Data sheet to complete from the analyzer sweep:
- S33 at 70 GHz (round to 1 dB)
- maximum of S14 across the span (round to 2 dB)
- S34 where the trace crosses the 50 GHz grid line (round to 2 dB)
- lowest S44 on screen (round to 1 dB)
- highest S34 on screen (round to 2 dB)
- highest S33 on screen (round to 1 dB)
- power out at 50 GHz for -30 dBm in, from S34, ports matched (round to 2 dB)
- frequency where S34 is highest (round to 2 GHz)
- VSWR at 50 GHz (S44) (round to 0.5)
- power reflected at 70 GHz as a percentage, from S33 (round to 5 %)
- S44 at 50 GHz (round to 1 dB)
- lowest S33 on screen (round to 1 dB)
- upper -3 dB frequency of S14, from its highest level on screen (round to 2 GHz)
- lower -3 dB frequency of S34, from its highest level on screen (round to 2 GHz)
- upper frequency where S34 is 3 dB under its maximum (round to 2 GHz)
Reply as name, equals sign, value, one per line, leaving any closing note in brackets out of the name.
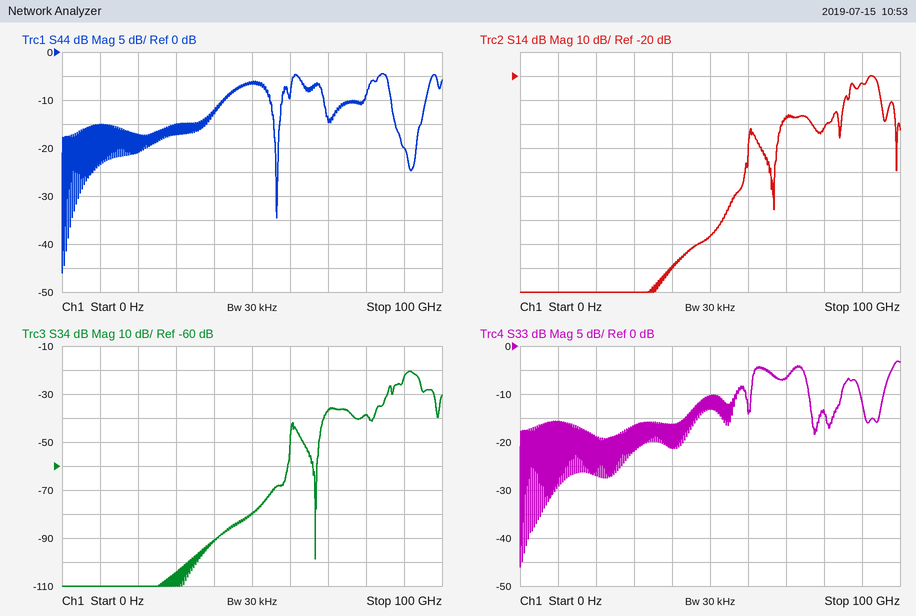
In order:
S33 at 70 GHz = -7 dB
maximum of S14 across the span = -20 dB
S34 where the trace crosses the 50 GHz grid line = -80 dB
lowest S44 on screen = -46 dB
highest S34 on screen = -20 dB
highest S33 on screen = -3 dB
power out at 50 GHz for -30 dBm in, from S34, ports matched = -110 dBm
frequency where S34 is highest = 92 GHz
VSWR at 50 GHz (S44) = 3.0
power reflected at 70 GHz as a percentage, from S33 = 20 %
S44 at 50 GHz = -6 dB
lowest S33 on screen = -46 dB
upper -3 dB frequency of S14, from its highest level on screen = 94 GHz
lower -3 dB frequency of S34, from its highest level on screen = 90 GHz
upper frequency where S34 is 3 dB under its maximum = 94 GHz
